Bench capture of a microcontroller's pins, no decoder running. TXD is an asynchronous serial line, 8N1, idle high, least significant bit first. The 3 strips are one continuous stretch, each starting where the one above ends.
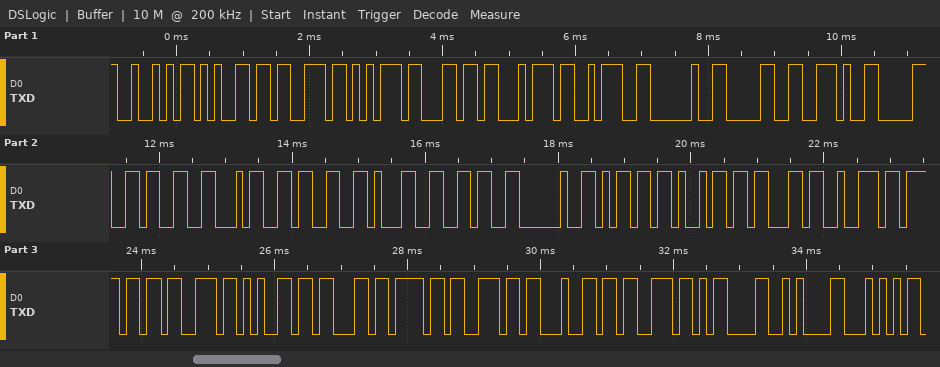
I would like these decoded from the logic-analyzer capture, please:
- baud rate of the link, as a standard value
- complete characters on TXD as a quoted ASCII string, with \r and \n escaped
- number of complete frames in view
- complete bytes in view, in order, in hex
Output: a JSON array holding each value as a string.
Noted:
["9600 baud", "\"Result: 0.034316 microseconds\\r\\nT\"", "32", "52 65 73 75 6C 74 3A 20 30 2E 30 33 34 33 31 36 20 6D 69 63 72 6F 73 65 63 6F 6E 64 73 0D 0A 54"]
